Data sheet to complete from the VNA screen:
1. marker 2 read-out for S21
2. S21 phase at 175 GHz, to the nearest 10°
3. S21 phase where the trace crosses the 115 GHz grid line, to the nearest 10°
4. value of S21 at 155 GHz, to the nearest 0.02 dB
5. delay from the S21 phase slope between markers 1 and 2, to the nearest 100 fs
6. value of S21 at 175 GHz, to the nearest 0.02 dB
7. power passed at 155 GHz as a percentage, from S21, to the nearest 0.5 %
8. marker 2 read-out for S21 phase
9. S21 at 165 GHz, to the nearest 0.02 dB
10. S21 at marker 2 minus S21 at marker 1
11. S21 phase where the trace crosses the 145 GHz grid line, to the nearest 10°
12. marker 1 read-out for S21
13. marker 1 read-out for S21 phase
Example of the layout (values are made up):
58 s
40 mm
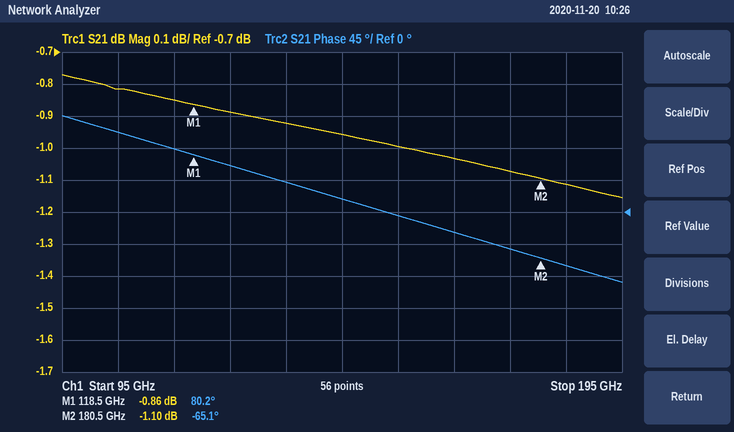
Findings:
-1.10 dB
-50°
90°
-1.00 dB
6.5 ps
-1.08 dB
79.5 %
-65.1°
-1.04 dB
-0.24 dB
20°
-0.86 dB
80.2°
